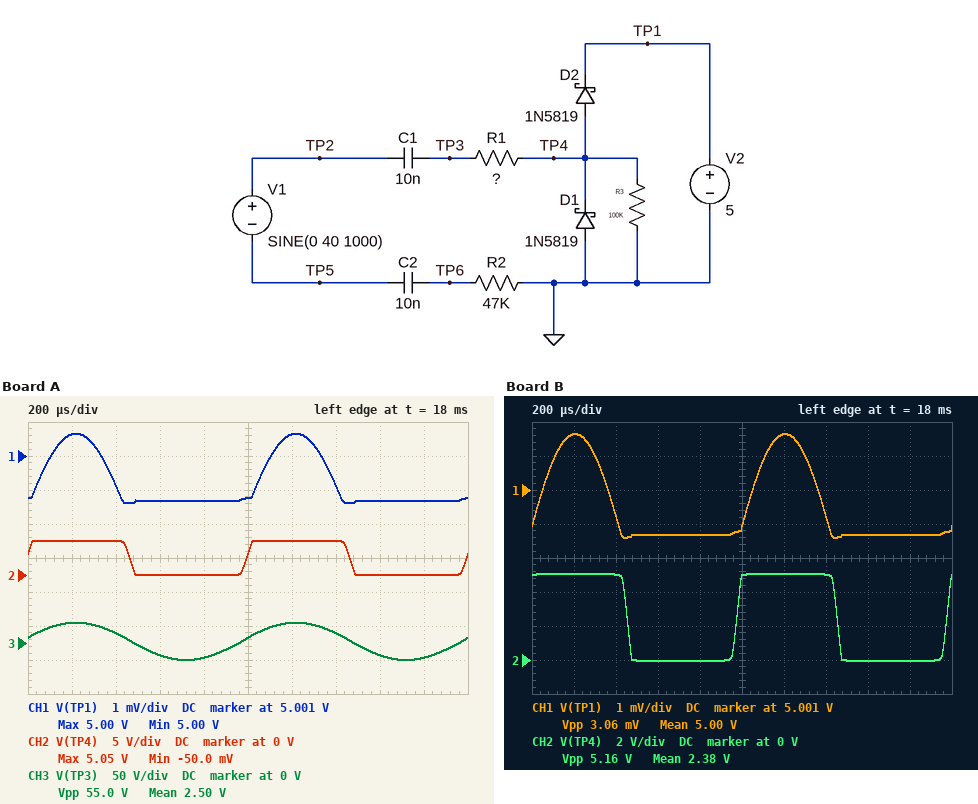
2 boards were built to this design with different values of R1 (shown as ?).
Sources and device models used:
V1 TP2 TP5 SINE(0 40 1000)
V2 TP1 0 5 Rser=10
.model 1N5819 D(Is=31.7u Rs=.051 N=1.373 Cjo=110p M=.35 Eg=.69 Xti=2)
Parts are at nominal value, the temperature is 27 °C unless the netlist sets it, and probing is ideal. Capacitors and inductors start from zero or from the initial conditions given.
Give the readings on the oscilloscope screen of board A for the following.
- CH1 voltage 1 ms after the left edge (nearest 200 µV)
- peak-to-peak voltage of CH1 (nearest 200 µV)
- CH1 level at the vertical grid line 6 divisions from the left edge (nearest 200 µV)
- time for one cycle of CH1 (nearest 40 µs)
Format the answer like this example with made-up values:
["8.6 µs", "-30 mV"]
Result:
["4.9998 V", "2.0 mV", "5.0016 V", "1.00 ms"]
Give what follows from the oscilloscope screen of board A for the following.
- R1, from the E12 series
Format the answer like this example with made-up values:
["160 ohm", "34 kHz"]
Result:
["100 kΩ"]
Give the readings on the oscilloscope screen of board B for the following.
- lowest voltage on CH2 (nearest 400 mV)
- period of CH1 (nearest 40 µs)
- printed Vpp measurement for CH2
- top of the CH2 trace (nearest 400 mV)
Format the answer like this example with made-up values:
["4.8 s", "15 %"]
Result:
["0 V", "1.00 ms", "5.16 V", "5.2 V"]
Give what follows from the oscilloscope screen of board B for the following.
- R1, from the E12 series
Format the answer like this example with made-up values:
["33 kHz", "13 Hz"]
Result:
["56 kΩ"]
